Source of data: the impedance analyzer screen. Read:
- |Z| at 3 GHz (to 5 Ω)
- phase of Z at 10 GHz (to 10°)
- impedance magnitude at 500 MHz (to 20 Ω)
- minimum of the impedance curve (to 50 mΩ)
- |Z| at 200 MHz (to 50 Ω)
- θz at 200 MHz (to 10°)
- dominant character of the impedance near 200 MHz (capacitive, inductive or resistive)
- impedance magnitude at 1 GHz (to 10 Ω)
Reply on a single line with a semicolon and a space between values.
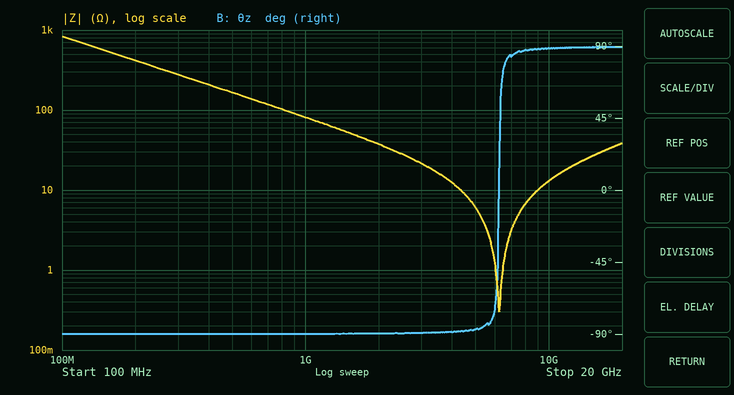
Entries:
20 Ω; 90°; 160 Ω; 300 mΩ; 400 Ω; -90°; capacitive; 80 Ω
